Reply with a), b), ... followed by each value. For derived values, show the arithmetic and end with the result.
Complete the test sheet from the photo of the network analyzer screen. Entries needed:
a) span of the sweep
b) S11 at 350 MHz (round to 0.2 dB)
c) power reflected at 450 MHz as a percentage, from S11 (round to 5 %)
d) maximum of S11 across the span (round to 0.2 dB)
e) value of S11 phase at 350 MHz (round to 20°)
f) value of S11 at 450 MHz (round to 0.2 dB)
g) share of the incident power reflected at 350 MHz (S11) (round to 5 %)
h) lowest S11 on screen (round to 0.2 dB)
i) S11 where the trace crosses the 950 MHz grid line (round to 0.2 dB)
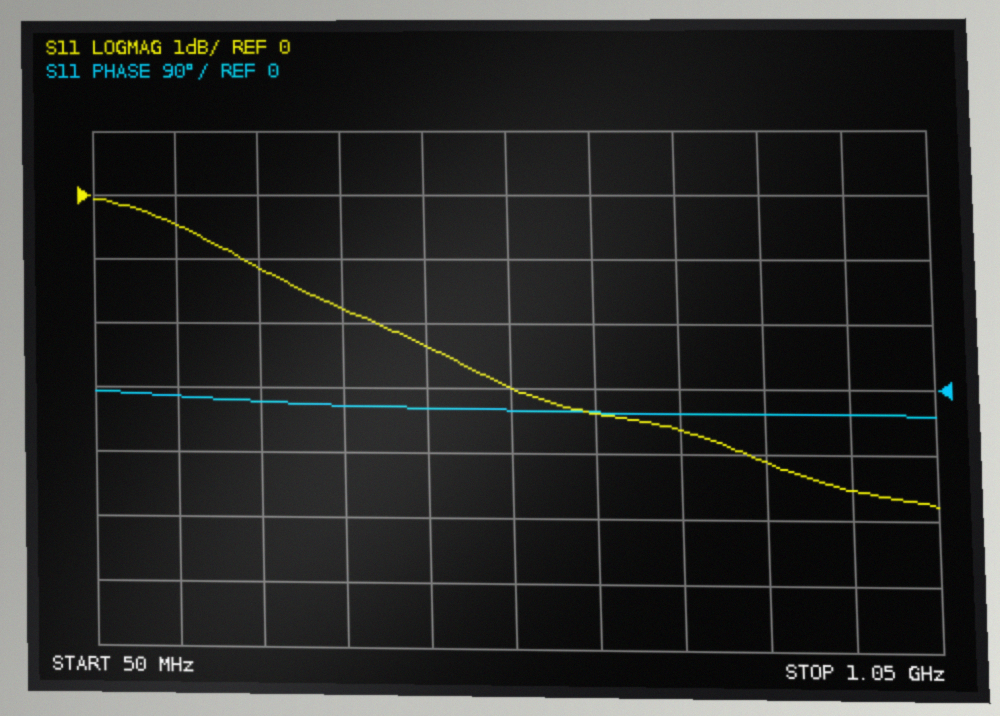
a) 1 GHz
b) -1.8 dB
c) 10^(-2.4/10) ≈ 57.5 %, so 60 % to the nearest 5 %
d) 0.0 dB
e) -20°
f) -2.4 dB
g) 10^(-1.8/10) ≈ 66.1 %, so 65 % to the nearest 5 %
h) -4.8 dB
i) -4.6 dB
